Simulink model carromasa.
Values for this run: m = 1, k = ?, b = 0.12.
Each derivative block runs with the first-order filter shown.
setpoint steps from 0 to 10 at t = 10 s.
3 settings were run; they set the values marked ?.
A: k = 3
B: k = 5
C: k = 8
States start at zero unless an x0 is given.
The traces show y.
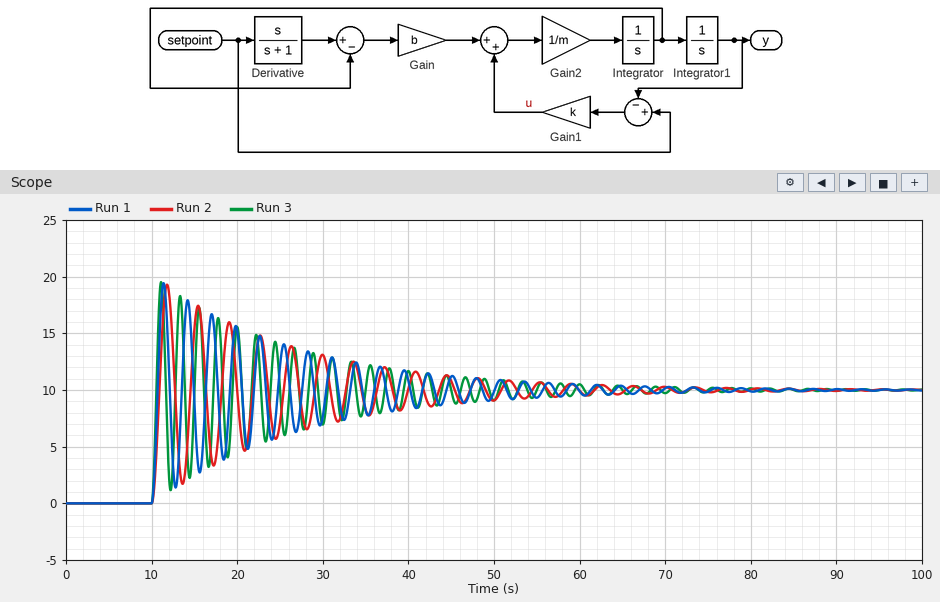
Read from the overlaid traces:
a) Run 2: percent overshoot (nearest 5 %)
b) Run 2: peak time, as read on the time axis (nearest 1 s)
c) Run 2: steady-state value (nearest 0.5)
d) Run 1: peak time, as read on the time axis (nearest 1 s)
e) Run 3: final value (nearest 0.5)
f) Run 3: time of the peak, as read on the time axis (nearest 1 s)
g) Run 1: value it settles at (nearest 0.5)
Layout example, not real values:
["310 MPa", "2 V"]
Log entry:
["95 %", "12 s", "10.0", "11 s", "10.0", "11 s", "10.0"]
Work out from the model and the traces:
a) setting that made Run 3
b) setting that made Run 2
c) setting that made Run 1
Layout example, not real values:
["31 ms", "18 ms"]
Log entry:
["C", "A", "B"]
